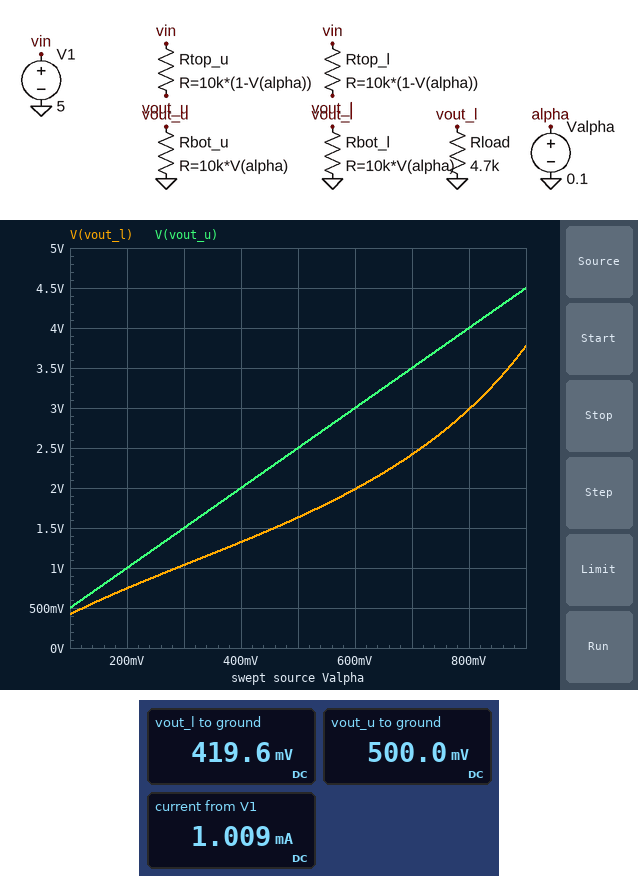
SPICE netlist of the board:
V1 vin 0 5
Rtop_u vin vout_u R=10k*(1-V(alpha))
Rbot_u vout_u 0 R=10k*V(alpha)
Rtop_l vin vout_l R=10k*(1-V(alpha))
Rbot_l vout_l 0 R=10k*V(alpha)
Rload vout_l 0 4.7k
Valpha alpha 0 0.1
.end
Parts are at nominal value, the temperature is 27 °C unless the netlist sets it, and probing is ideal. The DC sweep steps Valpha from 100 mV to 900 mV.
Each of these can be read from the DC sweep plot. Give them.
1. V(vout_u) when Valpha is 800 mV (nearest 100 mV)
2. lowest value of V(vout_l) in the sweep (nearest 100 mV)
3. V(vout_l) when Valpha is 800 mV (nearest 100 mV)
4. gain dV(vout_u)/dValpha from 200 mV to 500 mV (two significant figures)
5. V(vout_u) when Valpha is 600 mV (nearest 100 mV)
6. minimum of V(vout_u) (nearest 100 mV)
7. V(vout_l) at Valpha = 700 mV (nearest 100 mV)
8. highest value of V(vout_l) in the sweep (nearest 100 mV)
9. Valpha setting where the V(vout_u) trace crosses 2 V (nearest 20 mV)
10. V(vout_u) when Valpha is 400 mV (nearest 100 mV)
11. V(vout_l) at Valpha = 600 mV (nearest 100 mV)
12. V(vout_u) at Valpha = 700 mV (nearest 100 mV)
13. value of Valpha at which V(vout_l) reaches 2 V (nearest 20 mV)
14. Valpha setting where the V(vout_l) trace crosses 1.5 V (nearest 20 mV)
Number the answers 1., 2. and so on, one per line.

1. 4.0 V
2. 400 mV
3. 3.0 V
4. 5.0 V/V
5. 3.0 V
6. 500 mV
7. 2.4 V
8. 3.8 V
9. 400 mV
10. 2.0 V
11. 2.0 V
12. 3.5 V
13. 600 mV
14. 460 mV
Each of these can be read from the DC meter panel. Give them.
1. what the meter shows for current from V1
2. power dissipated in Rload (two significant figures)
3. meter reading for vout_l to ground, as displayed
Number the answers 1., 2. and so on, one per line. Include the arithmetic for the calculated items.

1. 1.009 mA
2. (419.6 mV)^2 / 4.7 kΩ = 37 µW
3. 419.6 mV
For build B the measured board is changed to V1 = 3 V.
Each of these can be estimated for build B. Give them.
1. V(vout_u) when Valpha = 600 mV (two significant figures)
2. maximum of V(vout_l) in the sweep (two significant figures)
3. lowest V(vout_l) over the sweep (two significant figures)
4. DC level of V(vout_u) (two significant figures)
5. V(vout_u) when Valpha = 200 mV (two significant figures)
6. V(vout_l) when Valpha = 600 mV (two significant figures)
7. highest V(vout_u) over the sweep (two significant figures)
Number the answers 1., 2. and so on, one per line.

1. 1.8 V
2. 2.3 V
3. 250 mV
4. 300 mV
5. 600 mV
6. 1.2 V
7. 2.7 V
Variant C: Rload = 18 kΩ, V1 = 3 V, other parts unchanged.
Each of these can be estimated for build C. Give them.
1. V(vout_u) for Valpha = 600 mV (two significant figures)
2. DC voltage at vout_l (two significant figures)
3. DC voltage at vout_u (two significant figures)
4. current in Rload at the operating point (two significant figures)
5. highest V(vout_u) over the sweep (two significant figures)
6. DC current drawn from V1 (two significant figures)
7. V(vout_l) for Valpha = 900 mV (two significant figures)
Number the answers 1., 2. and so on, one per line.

1. 1.8 V
2. 290 mV
3. 300 mV
4. 16 µA
5. 2.7 V
6. 600 µA
7. 2.6 V
